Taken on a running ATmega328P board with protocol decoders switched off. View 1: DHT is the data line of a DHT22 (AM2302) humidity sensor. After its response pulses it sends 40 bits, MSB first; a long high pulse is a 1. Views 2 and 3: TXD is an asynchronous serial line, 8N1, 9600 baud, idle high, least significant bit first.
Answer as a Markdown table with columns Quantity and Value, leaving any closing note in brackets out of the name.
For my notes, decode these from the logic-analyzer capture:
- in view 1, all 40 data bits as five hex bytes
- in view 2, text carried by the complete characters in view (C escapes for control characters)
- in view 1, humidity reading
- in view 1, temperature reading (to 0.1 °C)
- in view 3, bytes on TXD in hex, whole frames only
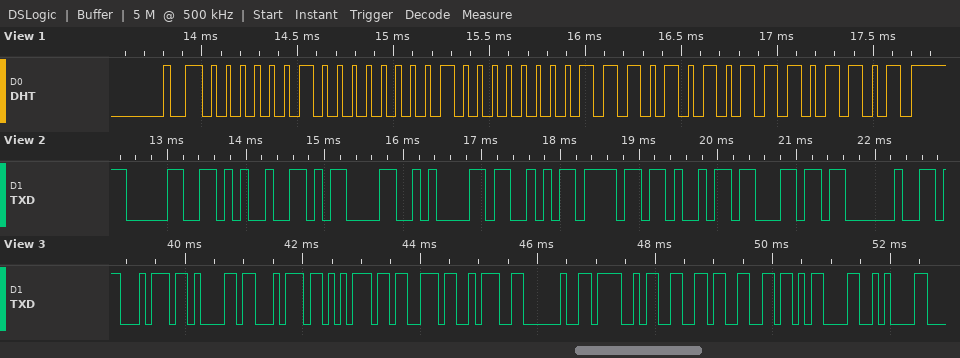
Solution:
| Quantity | Value |
|---|---|
| in view 1, all 40 data bits as five hex bytes | 02 01 00 EA ED |
| in view 2, text carried by the complete characters in view | "0%\r\nSoil " |
| in view 1, humidity reading | 51.3 % |
| in view 1, temperature reading | 23.4 °C |
| in view 3, bytes on TXD in hex, whole frames only | 74 61 74 75 73 3A 20 4F 66 66 0D 0A |
